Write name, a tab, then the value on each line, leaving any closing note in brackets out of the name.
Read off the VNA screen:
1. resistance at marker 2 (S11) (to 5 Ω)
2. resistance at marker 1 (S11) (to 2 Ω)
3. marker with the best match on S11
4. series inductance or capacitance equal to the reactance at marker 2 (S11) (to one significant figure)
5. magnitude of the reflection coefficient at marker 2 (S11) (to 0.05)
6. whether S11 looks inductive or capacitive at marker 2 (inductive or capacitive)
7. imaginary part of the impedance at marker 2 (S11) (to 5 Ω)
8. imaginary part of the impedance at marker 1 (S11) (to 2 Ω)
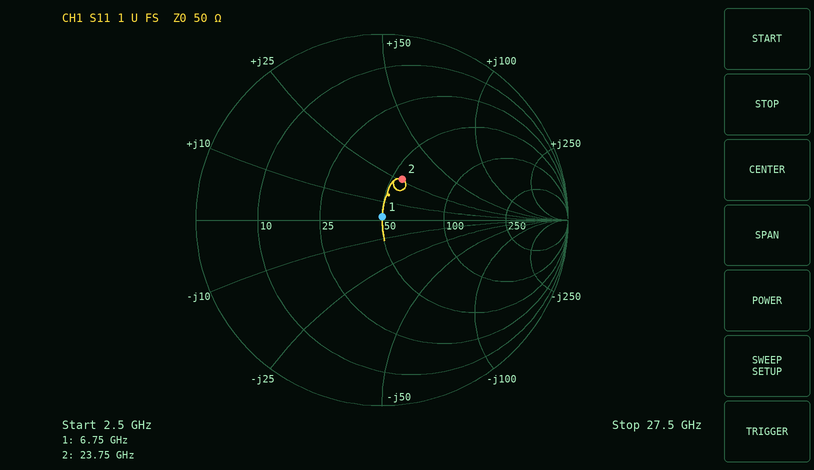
resistance at marker 2 (S11)	55 Ω
resistance at marker 1 (S11)	50 Ω
marker with the best match on S11	marker 1
series inductance or capacitance equal to the reactance at marker 2 (S11)	200 pH
magnitude of the reflection coefficient at marker 2 (S11)	0.25
whether S11 looks inductive or capacitive at marker 2	inductive
imaginary part of the impedance at marker 2 (S11)	+25 Ω
imaginary part of the impedance at marker 1 (S11)	+2 Ω
